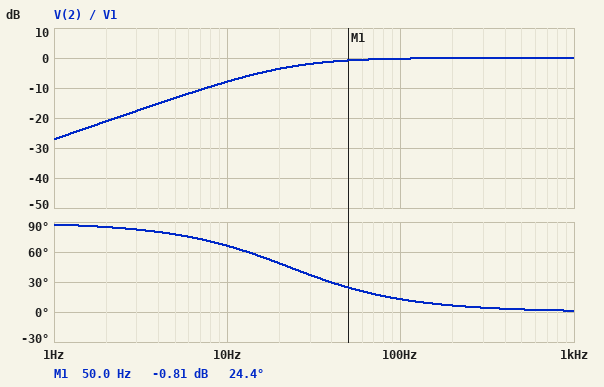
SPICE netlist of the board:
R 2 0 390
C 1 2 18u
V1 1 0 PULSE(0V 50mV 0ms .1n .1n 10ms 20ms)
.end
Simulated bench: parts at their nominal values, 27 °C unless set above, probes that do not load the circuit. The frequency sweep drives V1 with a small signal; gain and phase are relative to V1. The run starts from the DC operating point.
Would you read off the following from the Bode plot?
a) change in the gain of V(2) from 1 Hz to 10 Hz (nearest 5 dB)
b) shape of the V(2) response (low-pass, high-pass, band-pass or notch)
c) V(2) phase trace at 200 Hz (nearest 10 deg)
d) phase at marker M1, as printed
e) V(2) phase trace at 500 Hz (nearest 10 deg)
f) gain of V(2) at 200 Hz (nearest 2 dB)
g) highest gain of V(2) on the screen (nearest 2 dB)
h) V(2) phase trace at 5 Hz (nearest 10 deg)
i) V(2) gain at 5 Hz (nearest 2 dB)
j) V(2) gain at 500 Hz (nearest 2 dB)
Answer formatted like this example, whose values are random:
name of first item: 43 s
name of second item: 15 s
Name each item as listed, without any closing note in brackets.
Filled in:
change in the gain of V(2) from 1 Hz to 10 Hz: 20 dB
shape of the V(2) response: high-pass
V(2) phase trace at 200 Hz: 10 deg
phase at marker M1, as printed: 24.4 deg
V(2) phase trace at 500 Hz: 0 deg
gain of V(2) at 200 Hz: 0 dB
highest gain of V(2) on the screen: 0 dB
V(2) phase trace at 5 Hz: 80 deg
V(2) gain at 5 Hz: -14 dB
V(2) gain at 500 Hz: 0 dB
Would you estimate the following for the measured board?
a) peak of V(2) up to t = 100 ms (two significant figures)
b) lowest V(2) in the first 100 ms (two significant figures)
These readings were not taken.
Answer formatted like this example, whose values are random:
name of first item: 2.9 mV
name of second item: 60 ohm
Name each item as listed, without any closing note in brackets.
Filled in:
peak of V(2) up to t = 100 ms: 50 mV
lowest V(2) in the first 100 ms: -40 mV
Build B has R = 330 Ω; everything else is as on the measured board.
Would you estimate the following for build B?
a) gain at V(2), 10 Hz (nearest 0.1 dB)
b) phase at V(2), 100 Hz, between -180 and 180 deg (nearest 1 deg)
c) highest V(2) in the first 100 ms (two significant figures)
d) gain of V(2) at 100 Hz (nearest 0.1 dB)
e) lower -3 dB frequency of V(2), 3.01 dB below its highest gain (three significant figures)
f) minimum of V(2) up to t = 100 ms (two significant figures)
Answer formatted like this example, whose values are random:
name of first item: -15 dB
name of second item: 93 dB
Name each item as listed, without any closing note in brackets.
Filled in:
gain at V(2), 10 Hz: -9.1 dB
phase at V(2), 100 Hz, between -180 and 180 deg: 15 deg
highest V(2) in the first 100 ms: 50 mV
gain of V(2) at 100 Hz: -0.3 dB
lower -3 dB frequency of V(2), 3.01 dB below its highest gain: 26.8 Hz
minimum of V(2) up to t = 100 ms: -42 mV
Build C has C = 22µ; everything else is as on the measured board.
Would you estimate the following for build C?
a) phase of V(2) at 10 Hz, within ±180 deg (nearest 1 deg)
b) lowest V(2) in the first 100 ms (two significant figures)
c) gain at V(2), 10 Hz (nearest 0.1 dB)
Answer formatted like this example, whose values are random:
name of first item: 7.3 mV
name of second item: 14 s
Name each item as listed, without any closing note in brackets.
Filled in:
phase of V(2) at 10 Hz, within ±180 deg: 62 deg
lowest V(2) in the first 100 ms: -38 mV
gain at V(2), 10 Hz: -6.5 dB
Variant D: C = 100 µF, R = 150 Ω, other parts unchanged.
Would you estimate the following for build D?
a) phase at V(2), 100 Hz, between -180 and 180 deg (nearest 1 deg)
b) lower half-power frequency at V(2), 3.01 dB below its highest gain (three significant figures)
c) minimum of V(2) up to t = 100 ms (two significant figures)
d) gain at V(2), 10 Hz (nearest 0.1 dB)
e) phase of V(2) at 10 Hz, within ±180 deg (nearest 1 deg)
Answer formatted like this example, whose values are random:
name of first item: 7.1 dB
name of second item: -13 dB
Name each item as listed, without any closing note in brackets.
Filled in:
phase at V(2), 100 Hz, between -180 and 180 deg: 6 deg
lower half-power frequency at V(2), 3.01 dB below its highest gain: 10.6 Hz
minimum of V(2) up to t = 100 ms: -33 mV
gain at V(2), 10 Hz: -3.3 dB
phase of V(2) at 10 Hz, within ±180 deg: 47 deg
